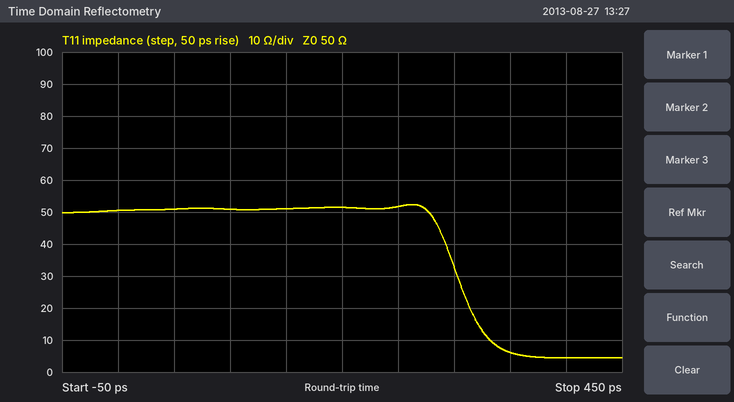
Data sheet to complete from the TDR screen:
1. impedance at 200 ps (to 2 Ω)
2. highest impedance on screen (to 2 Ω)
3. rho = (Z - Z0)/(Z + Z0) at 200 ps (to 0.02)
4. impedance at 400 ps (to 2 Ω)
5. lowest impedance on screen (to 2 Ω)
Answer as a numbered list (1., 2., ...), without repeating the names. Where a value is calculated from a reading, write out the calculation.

1. 52 Ω
2. 52 Ω
3. (52 − 50)/(52 + 50) ≈ +0.02
4. 4 Ω
5. 4 Ω
